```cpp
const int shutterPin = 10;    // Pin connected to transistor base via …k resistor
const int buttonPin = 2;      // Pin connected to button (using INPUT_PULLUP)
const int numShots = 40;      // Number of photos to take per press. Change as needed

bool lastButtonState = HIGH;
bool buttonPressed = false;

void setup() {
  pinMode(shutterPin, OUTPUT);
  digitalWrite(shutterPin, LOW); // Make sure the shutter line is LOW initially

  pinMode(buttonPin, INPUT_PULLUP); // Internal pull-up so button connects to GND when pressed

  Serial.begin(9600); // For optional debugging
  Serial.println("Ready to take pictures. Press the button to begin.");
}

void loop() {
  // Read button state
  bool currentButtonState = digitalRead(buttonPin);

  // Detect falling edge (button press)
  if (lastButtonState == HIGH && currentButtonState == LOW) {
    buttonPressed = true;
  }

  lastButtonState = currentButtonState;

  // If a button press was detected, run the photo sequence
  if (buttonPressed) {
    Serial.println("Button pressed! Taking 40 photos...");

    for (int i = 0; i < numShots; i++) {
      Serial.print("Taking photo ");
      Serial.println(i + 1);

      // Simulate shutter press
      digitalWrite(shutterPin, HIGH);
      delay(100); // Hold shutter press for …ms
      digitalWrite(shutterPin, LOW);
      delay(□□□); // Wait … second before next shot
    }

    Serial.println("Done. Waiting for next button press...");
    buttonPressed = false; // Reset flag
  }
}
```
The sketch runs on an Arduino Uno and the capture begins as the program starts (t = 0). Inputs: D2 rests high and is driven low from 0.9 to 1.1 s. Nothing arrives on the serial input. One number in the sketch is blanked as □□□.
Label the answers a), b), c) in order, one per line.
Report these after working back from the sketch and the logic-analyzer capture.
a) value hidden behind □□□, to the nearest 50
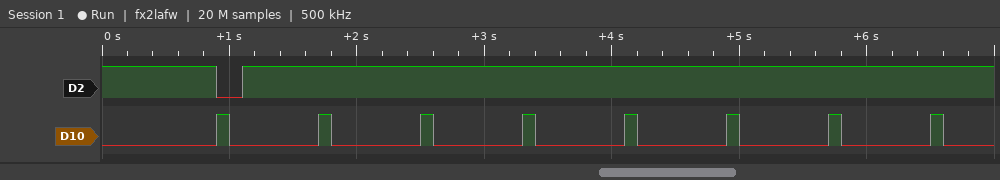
a) 700
